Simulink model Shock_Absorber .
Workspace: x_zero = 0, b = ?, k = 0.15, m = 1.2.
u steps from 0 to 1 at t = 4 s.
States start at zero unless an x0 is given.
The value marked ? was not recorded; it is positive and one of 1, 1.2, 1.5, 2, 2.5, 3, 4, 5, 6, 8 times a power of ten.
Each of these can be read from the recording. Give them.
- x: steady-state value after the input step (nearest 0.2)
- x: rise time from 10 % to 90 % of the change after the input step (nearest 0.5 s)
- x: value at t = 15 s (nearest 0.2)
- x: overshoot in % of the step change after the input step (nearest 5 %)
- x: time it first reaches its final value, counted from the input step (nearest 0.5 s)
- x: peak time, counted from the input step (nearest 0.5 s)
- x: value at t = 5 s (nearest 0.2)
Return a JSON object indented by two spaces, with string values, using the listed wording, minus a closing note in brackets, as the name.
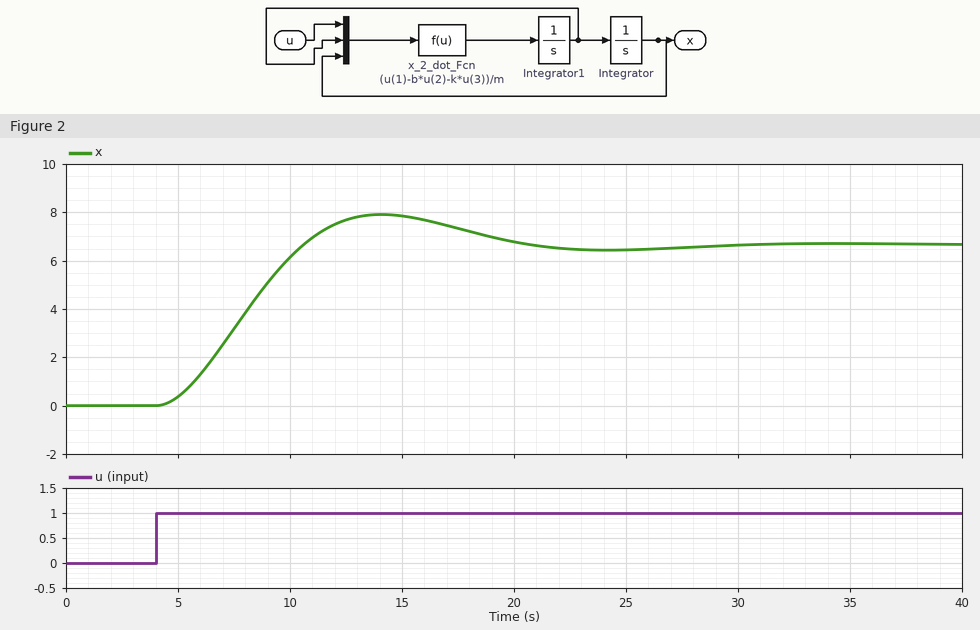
{
  "x: steady-state value after the input step": "6.6",
  "x: rise time from 10 % to 90 % of the change after the input step": "4.5 s",
  "x: value at t = 15 s": "7.8",
  "x: overshoot in % of the step change after the input step": "20 %",
  "x: time it first reaches its final value, counted from the input step": "6.5 s",
  "x: peak time, counted from the input step": "10.0 s",
  "x: value at t = 5 s": "0.4"
}
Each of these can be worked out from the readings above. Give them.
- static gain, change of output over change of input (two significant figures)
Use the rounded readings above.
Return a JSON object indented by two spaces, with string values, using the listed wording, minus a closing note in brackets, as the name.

{
  "static gain, change of output over change of input": "6.6"
}
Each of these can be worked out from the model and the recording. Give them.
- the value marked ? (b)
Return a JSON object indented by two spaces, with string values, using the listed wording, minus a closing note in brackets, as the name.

{
  "the value marked ?": "0.4"
}
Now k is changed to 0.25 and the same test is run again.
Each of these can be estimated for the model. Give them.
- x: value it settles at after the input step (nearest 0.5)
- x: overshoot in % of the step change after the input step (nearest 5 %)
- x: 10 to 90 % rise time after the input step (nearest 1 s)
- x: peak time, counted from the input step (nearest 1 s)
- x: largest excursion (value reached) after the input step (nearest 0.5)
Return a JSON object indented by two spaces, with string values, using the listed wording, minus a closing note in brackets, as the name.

{
  "x: value it settles at after the input step": "4.0",
  "x: overshoot in % of the step change after the input step": "30 %",
  "x: 10 to 90 % rise time after the input step": "3 s",
  "x: peak time, counted from the input step": "7 s",
  "x: largest excursion (value reached) after the input step": "5.0"
}
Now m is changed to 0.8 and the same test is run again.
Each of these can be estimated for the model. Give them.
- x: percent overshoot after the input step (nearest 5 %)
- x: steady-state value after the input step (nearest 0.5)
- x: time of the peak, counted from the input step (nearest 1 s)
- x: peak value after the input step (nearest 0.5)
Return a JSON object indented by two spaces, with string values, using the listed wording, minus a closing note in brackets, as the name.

{
  "x: percent overshoot after the input step": "10 %",
  "x: steady-state value after the input step": "6.5",
  "x: time of the peak, counted from the input step": "9 s",
  "x: peak value after the input step": "7.5"
}
